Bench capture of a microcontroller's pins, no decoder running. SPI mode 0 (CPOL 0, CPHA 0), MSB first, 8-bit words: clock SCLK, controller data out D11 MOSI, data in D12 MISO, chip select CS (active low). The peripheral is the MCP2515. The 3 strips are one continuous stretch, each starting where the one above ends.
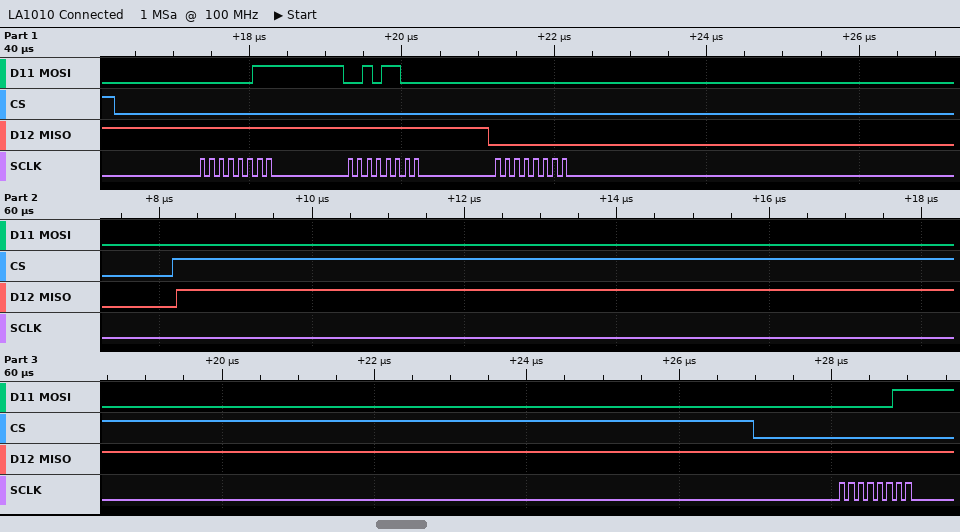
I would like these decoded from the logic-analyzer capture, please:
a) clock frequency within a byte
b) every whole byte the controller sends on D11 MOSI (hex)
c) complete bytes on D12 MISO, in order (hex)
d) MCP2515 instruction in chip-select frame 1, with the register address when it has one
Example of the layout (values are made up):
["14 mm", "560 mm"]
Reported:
["8 MHz", "0x03 0x2C 0x00 0x03", "0xFF 0xFF 0x00 0xFF", "READ 0x2C"]
